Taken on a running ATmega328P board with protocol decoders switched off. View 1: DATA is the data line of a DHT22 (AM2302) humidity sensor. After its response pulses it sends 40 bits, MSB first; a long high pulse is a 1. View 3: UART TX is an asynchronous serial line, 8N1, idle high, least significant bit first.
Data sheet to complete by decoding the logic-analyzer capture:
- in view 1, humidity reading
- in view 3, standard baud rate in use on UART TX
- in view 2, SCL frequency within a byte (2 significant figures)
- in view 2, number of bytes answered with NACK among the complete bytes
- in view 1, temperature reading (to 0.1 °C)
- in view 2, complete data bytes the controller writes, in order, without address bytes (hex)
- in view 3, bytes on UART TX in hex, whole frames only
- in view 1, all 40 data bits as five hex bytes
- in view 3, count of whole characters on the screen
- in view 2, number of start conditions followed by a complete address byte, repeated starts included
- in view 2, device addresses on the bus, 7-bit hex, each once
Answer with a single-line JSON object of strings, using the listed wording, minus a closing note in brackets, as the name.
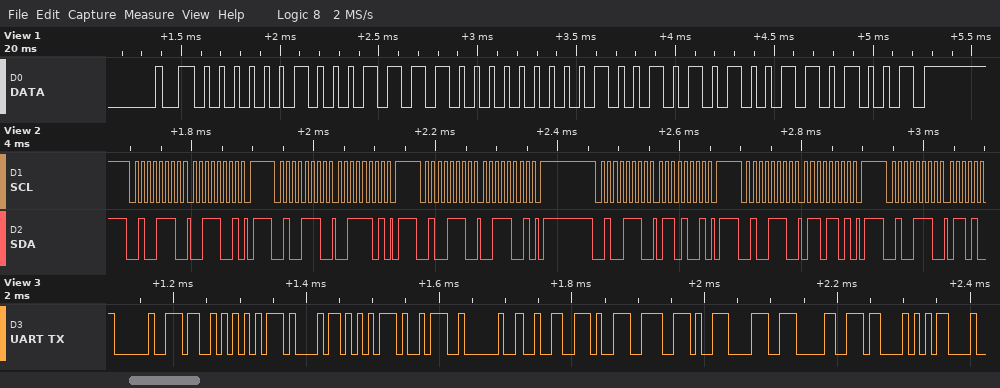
{"in view 1, humidity reading": "57.2 %", "in view 3, standard baud rate in use on UART TX": "115200 baud", "in view 2, SCL frequency within a byte": "100 kHz", "in view 2, number of bytes answered with NACK among the complete bytes": "0", "in view 1, temperature reading": "29.8 °C", "in view 2, complete data bytes the controller writes, in order, without address bytes": "39 3D 39 69 6D", "in view 3, bytes on UART TX in hex, whole frames only": "0x20 0x53 0x75 0x68 0x75 0x3A 0x20 0x32 0x39 0x2E 0x38 0x30 0x43 0x0D", "in view 1, all 40 data bits as five hex bytes": "02 3C 01 2A 69", "in view 3, count of whole characters on the screen": "14", "in view 2, number of start conditions followed by a complete address byte, repeated starts included": "6", "in view 2, device addresses on the bus, 7-bit hex, each once": "0x27"}
